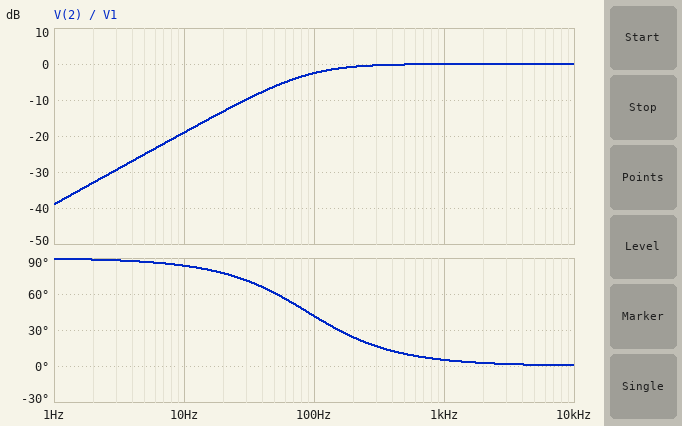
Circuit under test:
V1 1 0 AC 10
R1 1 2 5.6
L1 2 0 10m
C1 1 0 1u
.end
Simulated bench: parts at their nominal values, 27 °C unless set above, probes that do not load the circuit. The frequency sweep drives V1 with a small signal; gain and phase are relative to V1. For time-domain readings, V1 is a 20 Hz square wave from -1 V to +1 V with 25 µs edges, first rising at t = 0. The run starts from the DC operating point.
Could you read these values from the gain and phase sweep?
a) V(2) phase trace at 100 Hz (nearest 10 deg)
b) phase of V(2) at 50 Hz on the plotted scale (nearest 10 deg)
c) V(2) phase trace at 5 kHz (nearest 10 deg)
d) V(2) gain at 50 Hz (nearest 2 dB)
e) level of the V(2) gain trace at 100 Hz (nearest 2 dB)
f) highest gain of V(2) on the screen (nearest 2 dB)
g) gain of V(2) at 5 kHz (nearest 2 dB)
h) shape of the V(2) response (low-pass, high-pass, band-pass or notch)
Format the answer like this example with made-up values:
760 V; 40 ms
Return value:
40 deg; 60 deg; 0 deg; -6 dB; -2 dB; 0 dB; 0 dB; high-pass
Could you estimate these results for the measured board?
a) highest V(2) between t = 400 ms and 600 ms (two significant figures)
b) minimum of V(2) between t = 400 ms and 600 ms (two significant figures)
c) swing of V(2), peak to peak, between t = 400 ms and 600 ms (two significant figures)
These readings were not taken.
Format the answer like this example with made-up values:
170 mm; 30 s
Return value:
2.0 V; -2.0 V; 4.0 V
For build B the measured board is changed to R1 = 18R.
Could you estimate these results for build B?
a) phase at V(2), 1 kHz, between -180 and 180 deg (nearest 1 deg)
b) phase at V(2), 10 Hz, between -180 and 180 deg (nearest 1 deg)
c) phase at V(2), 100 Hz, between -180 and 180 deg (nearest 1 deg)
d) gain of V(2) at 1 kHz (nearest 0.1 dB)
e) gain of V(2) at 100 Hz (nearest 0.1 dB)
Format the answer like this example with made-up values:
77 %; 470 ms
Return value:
16 deg; 88 deg; 71 deg; -0.3 dB; -9.6 dB
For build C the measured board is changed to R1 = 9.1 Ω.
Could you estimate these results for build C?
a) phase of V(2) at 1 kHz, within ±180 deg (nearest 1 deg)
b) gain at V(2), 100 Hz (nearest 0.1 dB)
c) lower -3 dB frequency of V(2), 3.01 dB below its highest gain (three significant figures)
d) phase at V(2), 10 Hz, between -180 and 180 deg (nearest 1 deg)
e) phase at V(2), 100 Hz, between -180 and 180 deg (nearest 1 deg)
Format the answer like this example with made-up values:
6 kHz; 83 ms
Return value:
8 deg; -4.9 dB; 145 Hz; 86 deg; 55 deg
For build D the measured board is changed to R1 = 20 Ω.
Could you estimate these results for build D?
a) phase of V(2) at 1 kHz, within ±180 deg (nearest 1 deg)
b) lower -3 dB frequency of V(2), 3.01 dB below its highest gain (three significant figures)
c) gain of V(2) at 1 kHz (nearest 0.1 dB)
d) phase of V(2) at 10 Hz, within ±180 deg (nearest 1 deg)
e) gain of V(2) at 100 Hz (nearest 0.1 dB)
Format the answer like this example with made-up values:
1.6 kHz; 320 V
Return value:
18 deg; 318 Hz; -0.4 dB; 88 deg; -10.5 dB
